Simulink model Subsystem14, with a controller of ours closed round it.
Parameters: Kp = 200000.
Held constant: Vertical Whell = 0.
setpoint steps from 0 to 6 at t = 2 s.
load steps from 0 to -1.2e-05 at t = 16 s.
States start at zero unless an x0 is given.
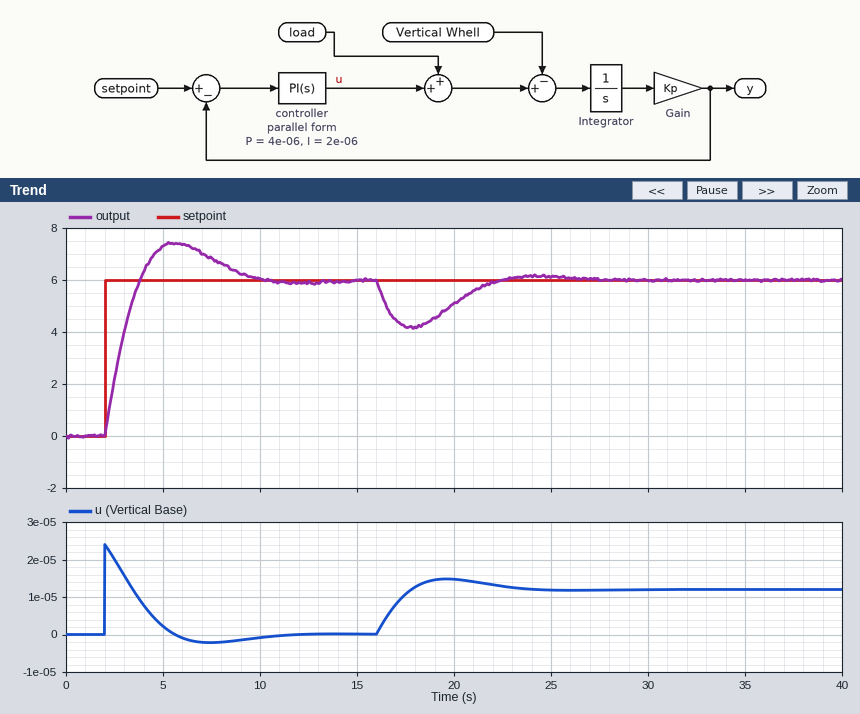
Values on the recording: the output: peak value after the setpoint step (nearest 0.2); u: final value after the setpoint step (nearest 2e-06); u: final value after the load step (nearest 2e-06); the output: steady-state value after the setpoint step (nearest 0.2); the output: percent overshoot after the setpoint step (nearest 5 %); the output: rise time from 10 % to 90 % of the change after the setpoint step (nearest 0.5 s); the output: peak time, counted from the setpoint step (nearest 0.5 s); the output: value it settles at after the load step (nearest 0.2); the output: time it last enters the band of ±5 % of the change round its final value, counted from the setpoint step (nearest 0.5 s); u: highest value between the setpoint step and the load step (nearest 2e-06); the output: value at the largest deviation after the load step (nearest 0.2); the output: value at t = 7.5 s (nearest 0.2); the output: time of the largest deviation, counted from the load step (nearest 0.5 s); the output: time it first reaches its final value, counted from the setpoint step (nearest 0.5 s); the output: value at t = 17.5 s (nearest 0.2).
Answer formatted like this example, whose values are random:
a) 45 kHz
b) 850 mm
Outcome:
a) 7.4
b) 0.000000
c) 0.000012
d) 6.0
e) 25 %
f) 1.5 s
g) 3.5 s
h) 6.0
i) 7.0 s
j) 0.000024
k) 4.2
l) 6.8
m) 2.0 s
n) 2.0 s
o) 4.2
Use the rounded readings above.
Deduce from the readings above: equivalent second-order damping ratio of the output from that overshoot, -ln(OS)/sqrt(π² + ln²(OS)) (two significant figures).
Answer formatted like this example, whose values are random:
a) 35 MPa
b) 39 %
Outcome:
a) 0.40
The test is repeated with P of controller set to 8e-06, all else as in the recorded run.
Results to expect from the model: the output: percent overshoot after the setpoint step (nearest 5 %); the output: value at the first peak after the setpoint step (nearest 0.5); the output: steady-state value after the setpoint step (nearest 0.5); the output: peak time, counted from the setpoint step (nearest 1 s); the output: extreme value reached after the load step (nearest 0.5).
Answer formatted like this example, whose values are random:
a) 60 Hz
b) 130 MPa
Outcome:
a) 10 %
b) 6.5
c) 6.0
d) 3 s
e) 5.0
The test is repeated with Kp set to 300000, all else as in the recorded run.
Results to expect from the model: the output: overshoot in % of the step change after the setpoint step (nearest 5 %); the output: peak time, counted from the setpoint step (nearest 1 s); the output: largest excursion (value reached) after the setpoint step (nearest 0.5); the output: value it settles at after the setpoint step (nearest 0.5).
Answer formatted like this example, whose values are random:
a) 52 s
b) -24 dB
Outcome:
a) 20 %
b) 3 s
c) 7.0
d) 6.0
